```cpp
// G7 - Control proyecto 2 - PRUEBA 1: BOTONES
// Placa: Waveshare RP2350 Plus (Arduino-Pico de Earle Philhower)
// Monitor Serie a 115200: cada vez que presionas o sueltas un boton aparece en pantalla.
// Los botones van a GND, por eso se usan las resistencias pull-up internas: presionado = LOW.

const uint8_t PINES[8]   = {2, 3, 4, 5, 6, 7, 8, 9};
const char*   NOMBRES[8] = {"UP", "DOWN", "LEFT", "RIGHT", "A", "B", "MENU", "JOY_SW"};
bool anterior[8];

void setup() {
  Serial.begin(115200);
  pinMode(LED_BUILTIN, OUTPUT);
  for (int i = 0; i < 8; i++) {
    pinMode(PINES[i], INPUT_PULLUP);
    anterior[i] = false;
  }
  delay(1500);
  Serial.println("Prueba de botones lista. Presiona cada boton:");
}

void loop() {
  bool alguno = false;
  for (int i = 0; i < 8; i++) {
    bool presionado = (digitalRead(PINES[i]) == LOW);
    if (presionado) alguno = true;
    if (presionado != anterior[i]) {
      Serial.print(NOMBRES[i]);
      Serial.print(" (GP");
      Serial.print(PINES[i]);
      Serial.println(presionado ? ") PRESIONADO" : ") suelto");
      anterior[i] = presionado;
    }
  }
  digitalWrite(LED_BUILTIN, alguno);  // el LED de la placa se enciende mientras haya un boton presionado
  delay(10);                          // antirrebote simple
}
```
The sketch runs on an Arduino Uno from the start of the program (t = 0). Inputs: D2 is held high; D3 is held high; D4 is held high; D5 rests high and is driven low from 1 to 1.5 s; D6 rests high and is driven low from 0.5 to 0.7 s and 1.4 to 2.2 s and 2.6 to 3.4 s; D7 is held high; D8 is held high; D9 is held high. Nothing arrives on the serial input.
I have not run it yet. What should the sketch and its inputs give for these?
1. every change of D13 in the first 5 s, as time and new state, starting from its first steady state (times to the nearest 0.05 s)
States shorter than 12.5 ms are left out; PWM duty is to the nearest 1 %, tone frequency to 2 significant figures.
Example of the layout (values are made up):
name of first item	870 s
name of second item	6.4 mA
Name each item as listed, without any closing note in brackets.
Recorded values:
every change of D13 in the first 5 s, as time and new state, starting from its first steady state	0 s low; 1.5 s high; 2.2 s low; 2.6 s high; 3.4 s low
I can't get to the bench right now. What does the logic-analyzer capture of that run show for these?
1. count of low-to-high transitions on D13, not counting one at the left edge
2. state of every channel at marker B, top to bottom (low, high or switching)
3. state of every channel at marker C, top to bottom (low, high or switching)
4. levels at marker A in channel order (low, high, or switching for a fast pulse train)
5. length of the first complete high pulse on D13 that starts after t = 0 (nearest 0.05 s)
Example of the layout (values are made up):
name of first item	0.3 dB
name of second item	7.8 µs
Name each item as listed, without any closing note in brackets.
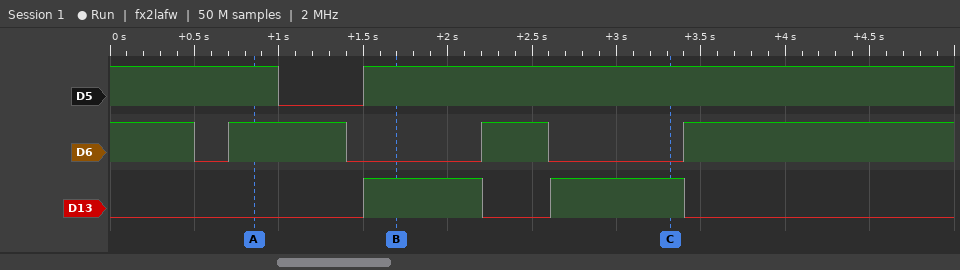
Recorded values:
count of low-to-high transitions on D13, not counting one at the left edge	2
state of every channel at marker B, top to bottom	D5 high, D6 low, D13 high
state of every channel at marker C, top to bottom	D5 high, D6 low, D13 high
levels at marker A in channel order	D5 high, D6 high, D13 low
length of the first complete high pulse on D13 that starts after t = 0	0.70 s
